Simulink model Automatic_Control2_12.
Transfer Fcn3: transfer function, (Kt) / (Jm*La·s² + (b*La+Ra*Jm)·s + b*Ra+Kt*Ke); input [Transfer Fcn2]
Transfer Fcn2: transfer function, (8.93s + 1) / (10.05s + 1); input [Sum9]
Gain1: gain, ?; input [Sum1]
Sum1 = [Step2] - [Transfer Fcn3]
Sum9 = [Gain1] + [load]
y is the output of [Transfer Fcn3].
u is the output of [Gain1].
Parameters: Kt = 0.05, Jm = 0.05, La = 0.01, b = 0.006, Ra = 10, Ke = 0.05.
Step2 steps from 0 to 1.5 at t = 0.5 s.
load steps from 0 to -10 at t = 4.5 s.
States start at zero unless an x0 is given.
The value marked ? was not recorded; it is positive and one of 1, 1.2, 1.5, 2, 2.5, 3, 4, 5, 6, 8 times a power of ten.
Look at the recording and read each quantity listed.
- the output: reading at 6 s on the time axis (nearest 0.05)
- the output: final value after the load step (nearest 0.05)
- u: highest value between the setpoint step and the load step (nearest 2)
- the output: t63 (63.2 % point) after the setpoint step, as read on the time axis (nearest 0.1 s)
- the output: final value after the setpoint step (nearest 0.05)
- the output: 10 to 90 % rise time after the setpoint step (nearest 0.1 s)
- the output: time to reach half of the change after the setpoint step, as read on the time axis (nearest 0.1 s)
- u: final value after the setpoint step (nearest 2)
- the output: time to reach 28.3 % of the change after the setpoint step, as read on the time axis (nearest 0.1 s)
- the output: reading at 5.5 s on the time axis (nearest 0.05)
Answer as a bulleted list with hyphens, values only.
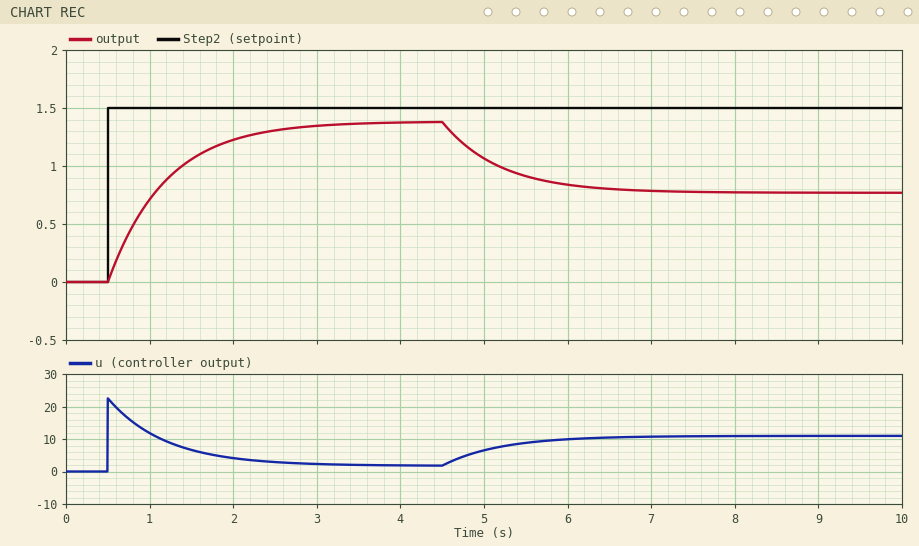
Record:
- 0.85
- 0.75
- 22
- 1.2 s
- 1.40
- 1.5 s
- 1.0 s
- 2
- 0.7 s
- 0.90
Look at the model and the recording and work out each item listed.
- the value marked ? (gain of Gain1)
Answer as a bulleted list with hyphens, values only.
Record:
- 15
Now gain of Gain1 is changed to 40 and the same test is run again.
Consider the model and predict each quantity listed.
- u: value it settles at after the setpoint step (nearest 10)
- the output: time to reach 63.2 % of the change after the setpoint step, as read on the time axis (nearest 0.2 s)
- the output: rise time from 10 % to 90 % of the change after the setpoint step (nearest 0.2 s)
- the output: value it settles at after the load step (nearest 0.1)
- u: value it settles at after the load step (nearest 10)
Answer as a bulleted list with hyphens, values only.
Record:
- 0
- 0.8 s
- 0.6 s
- 1.2
- 10
